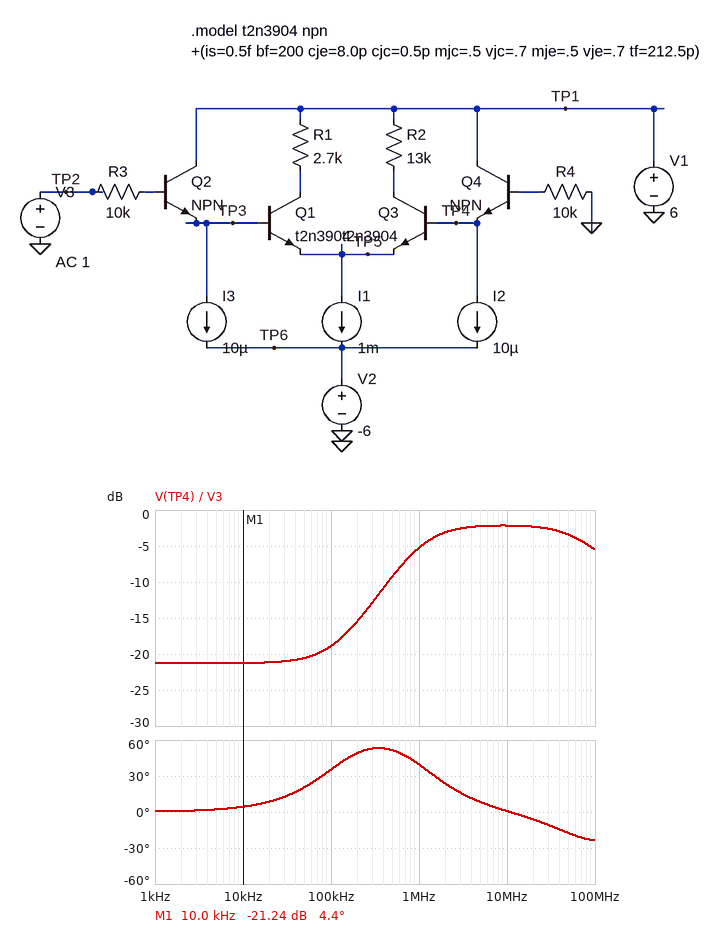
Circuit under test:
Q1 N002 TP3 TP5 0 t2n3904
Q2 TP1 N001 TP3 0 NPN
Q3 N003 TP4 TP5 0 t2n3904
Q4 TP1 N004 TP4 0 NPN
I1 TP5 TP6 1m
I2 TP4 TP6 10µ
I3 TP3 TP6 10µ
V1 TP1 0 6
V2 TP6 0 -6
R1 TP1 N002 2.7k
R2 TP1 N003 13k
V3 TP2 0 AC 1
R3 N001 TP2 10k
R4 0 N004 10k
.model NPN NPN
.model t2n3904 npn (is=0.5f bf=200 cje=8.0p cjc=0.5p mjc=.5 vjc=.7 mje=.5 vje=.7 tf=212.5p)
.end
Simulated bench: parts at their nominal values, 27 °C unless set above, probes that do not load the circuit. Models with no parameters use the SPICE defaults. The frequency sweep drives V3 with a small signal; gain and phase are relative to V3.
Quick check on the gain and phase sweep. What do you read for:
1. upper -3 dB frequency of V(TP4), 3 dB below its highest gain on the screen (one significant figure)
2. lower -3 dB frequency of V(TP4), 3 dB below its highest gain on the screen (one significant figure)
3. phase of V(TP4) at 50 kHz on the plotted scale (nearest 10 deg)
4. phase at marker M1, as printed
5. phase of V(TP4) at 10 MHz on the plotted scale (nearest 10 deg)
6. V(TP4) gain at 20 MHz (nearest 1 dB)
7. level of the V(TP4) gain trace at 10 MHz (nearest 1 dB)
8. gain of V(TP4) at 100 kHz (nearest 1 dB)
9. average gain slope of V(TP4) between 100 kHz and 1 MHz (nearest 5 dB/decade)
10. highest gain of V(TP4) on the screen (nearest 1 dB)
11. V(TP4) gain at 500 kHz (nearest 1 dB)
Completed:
90 MHz
1 MHz
20 deg
4.4 deg
0 deg
-2 dB
-2 dB
-19 dB
15 dB/decade
-2 dB
-9 dB
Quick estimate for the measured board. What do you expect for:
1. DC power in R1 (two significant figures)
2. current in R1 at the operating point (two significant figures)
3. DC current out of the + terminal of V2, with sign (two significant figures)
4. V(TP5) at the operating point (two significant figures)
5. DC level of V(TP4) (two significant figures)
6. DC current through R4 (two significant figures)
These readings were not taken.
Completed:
670 µW
500 µA
-1.0 mA
-1.4 V
-660 mV
120 nA
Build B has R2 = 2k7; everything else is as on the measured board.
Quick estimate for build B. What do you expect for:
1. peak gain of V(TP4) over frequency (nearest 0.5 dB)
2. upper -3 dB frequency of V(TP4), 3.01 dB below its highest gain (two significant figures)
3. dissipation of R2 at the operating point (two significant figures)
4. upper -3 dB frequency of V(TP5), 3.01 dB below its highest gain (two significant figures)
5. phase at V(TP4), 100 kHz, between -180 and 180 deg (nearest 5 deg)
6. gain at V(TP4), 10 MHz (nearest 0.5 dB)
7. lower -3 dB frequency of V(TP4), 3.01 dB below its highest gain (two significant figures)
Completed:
-6.0 dB
330 MHz
670 µW
310 MHz
10 deg
-6.5 dB
2.8 MHz
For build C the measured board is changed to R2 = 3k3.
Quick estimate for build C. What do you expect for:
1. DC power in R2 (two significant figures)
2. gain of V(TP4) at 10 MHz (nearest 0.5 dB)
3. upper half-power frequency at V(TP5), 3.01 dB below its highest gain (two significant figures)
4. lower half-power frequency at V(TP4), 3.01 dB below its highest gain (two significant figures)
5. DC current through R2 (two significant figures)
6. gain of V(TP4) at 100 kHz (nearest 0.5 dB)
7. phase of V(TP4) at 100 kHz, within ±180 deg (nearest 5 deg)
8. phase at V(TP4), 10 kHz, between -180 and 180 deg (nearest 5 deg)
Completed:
820 µW
-6.0 dB
280 MHz
2.7 MHz
500 µA
-21.0 dB
10 deg
0 deg
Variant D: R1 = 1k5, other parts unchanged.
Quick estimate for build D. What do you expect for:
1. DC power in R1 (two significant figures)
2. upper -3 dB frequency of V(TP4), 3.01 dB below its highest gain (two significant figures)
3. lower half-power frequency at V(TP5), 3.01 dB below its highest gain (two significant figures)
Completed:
370 µW
100 MHz
540 kHz
